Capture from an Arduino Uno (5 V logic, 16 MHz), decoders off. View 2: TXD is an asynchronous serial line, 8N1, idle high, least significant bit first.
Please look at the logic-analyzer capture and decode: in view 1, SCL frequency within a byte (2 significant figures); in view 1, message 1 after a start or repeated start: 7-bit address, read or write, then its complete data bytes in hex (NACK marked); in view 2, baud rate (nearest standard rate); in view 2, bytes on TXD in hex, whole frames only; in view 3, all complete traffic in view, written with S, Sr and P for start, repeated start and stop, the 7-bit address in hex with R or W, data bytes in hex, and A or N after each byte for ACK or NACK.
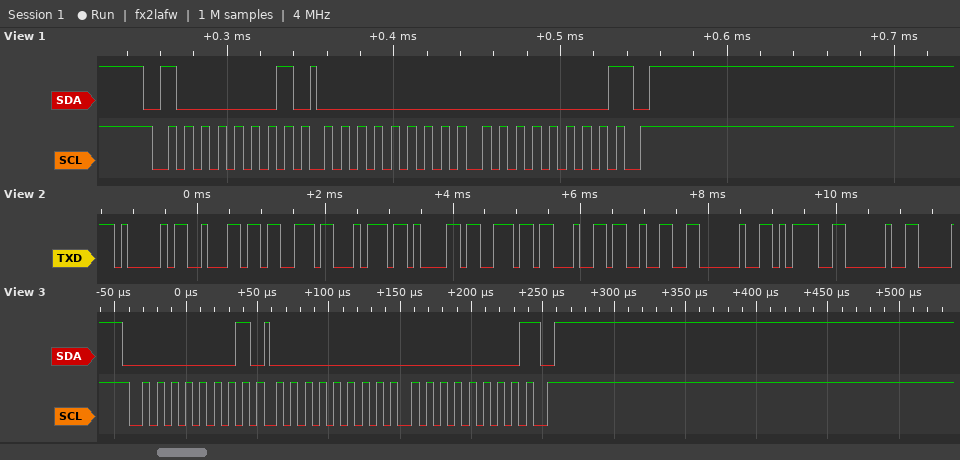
100 kHz
0x40 read: 00 00 NACK
9600 baud
41 62 73 74 61 6E 64 32 20 3D 20
S 00R A 00 A 00 N P
